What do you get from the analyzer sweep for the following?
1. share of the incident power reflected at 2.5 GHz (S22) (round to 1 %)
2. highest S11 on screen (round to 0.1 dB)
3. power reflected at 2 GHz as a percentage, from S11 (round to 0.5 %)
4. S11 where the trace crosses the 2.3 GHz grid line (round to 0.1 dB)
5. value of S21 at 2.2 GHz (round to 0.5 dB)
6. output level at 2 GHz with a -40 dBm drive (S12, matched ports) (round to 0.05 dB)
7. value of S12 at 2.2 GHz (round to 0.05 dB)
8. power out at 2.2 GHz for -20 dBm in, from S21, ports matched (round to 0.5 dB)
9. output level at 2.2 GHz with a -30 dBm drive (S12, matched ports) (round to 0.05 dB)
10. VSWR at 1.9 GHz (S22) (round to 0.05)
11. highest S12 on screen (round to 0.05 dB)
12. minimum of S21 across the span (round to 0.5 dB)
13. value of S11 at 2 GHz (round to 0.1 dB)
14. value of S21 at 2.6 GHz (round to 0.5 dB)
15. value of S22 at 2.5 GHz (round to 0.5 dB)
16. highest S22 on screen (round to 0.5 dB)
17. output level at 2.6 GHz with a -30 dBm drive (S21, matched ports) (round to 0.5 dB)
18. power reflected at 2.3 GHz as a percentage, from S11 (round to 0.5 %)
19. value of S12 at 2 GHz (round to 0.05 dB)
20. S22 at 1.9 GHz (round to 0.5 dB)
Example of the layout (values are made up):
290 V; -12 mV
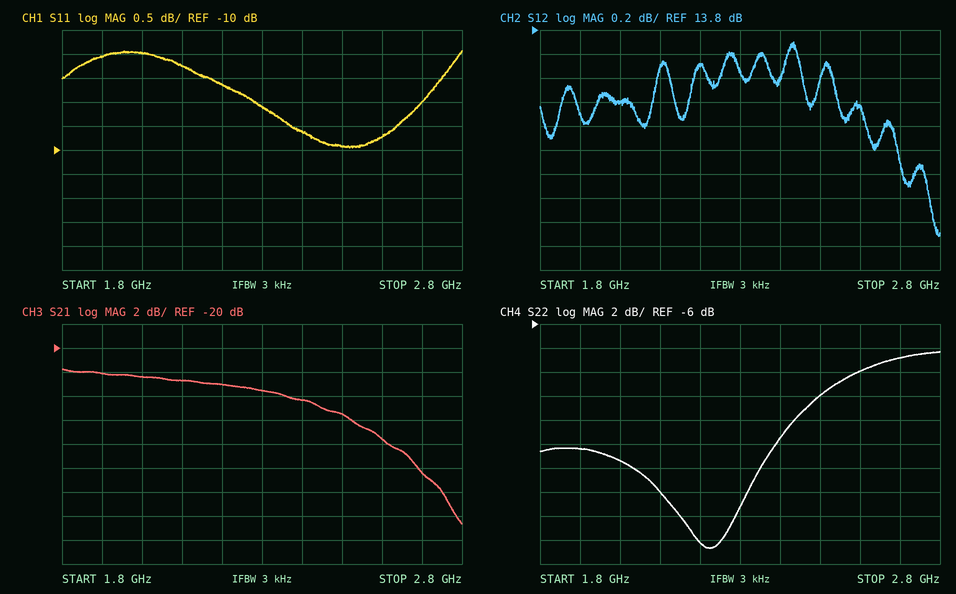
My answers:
6 %; -7.9 dB; 16.0 %; -9.1 dB; -23.0 dB; -26.80 dBm; 13.50 dB; -43.0 dBm; -16.50 dBm; 1.35; 13.70 dB; -34.5 dB; -8.0 dB; -27.5 dB; -12.0 dB; -8.5 dB; -57.5 dBm; 12.5 %; 13.20 dB; -16.5 dB
